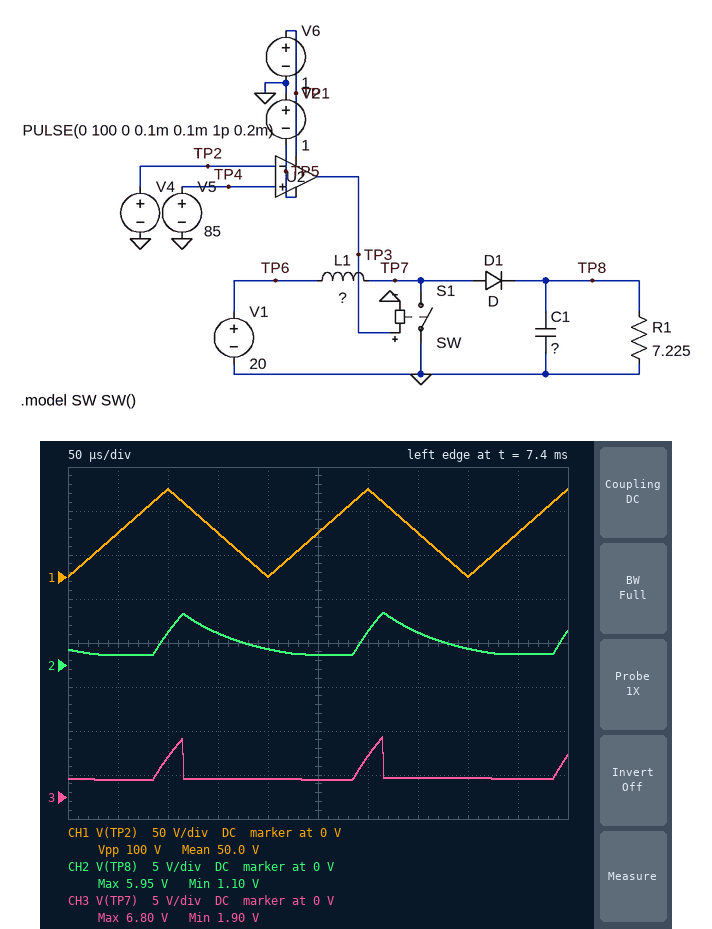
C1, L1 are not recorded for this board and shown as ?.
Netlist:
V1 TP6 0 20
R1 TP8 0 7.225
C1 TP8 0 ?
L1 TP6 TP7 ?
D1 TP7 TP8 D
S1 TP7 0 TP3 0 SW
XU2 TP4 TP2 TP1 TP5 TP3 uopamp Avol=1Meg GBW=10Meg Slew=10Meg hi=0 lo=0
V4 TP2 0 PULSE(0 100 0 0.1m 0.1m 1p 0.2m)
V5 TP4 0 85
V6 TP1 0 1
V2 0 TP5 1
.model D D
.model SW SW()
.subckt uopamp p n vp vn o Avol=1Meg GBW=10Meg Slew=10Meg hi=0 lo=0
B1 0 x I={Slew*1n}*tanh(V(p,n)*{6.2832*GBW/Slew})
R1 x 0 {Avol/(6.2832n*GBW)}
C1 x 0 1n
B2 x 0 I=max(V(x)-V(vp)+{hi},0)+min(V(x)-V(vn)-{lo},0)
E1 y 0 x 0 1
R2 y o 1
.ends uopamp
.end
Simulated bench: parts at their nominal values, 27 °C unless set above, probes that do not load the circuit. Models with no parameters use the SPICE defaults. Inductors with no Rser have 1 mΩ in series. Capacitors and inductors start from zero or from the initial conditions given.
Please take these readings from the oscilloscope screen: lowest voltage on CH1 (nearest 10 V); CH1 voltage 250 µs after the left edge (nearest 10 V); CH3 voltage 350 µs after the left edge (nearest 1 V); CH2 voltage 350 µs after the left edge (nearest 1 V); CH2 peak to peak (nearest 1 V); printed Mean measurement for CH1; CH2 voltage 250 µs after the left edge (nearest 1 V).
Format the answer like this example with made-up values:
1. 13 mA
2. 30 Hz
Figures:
1. 0 V
2. 50 V
3. 2 V
4. 4 V
5. 5 V
6. 50.0 V
7. 1 V
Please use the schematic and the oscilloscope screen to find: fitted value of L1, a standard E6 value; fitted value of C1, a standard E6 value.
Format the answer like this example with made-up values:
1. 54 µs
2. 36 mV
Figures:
1. 68 mH
2. 10 µF
